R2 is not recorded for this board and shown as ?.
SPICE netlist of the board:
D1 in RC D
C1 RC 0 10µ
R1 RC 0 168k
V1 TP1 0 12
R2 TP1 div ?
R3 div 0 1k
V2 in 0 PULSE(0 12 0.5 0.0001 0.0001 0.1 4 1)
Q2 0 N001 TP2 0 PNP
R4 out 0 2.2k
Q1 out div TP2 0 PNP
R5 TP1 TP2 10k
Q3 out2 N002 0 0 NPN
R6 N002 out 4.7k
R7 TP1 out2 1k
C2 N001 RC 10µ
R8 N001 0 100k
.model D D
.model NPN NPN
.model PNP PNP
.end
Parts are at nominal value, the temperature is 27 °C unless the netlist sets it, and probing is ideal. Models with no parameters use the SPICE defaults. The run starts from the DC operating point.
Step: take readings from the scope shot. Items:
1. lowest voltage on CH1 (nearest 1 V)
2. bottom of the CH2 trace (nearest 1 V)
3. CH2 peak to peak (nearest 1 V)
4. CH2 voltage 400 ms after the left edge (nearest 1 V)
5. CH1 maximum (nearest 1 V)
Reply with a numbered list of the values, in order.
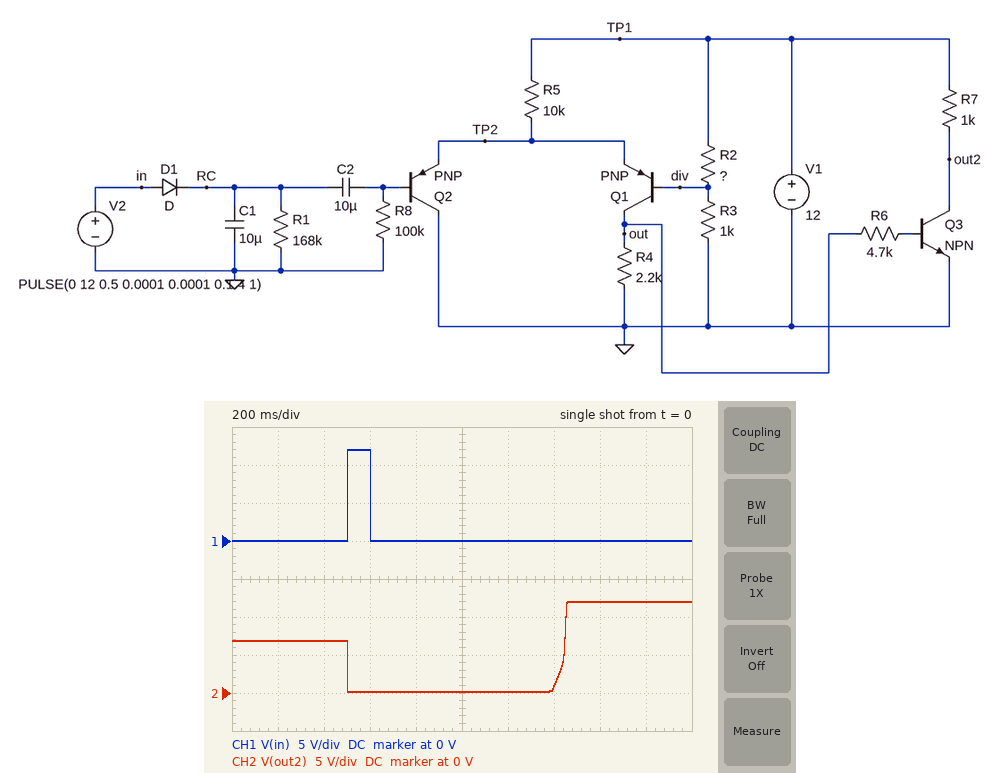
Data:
1. 0 V
2. 0 V
3. 12 V
4. 7 V
5. 12 V
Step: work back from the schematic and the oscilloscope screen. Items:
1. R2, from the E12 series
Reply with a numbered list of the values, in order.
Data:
1. 22 kΩ
